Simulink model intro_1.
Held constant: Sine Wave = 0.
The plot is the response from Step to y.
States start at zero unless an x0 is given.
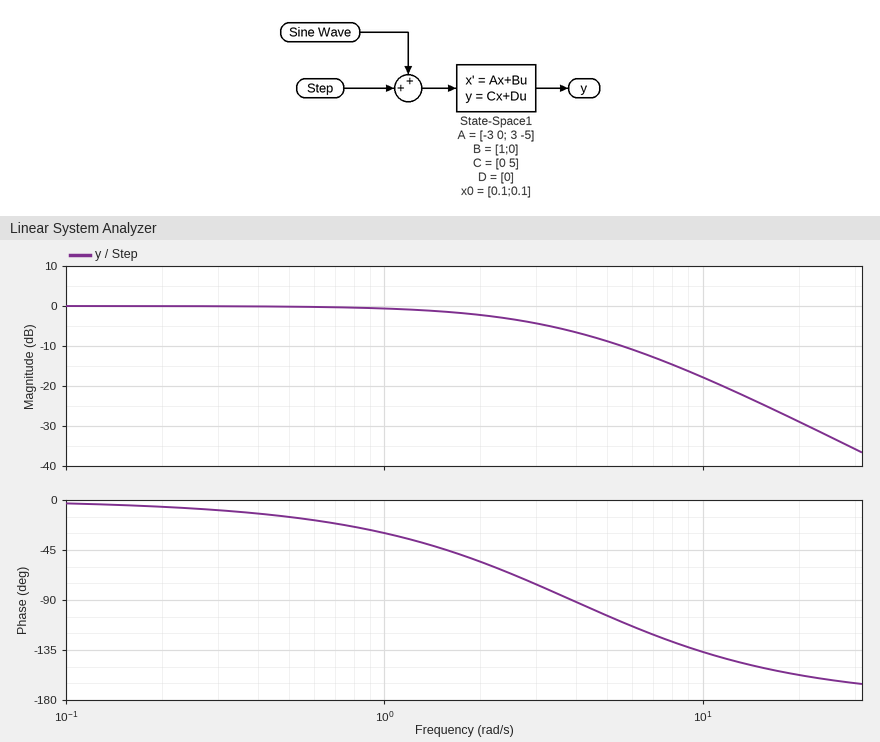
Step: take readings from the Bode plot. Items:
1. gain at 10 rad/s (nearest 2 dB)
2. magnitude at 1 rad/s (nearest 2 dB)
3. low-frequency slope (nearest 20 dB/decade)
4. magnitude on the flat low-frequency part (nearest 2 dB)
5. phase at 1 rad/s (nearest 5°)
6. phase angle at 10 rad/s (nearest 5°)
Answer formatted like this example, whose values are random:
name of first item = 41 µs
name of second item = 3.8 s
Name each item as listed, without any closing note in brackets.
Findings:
gain at 10 rad/s = -18 dB
magnitude at 1 rad/s = 0 dB
low-frequency slope = 0 dB/decade
magnitude on the flat low-frequency part = 0 dB
phase at 1 rad/s = -30°
phase angle at 10 rad/s = -135°
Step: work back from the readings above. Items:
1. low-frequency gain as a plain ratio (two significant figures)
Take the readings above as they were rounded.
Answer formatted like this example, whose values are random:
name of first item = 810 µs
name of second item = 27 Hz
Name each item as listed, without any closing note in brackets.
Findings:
low-frequency gain as a plain ratio = 1.0
